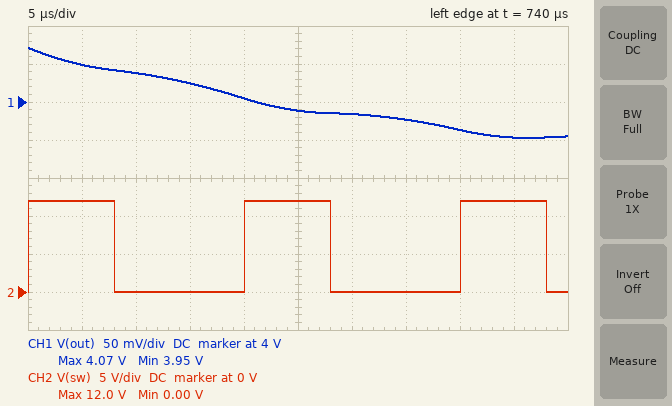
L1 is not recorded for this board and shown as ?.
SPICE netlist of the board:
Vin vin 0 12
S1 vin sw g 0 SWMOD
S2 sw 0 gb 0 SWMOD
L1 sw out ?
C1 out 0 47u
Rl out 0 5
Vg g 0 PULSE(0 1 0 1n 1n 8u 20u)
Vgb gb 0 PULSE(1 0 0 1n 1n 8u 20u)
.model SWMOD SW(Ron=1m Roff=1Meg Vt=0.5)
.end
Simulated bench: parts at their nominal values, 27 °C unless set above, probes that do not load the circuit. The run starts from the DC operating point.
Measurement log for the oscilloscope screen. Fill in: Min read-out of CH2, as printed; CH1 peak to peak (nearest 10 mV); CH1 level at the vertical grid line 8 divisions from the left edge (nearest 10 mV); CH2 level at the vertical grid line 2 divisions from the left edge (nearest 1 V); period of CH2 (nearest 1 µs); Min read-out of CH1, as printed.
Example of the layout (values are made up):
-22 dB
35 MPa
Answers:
0.00 V
120 mV
3.96 V
0 V
20 µs
3.95 V
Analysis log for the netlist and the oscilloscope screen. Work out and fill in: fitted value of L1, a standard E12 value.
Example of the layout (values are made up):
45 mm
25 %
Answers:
330 µH
